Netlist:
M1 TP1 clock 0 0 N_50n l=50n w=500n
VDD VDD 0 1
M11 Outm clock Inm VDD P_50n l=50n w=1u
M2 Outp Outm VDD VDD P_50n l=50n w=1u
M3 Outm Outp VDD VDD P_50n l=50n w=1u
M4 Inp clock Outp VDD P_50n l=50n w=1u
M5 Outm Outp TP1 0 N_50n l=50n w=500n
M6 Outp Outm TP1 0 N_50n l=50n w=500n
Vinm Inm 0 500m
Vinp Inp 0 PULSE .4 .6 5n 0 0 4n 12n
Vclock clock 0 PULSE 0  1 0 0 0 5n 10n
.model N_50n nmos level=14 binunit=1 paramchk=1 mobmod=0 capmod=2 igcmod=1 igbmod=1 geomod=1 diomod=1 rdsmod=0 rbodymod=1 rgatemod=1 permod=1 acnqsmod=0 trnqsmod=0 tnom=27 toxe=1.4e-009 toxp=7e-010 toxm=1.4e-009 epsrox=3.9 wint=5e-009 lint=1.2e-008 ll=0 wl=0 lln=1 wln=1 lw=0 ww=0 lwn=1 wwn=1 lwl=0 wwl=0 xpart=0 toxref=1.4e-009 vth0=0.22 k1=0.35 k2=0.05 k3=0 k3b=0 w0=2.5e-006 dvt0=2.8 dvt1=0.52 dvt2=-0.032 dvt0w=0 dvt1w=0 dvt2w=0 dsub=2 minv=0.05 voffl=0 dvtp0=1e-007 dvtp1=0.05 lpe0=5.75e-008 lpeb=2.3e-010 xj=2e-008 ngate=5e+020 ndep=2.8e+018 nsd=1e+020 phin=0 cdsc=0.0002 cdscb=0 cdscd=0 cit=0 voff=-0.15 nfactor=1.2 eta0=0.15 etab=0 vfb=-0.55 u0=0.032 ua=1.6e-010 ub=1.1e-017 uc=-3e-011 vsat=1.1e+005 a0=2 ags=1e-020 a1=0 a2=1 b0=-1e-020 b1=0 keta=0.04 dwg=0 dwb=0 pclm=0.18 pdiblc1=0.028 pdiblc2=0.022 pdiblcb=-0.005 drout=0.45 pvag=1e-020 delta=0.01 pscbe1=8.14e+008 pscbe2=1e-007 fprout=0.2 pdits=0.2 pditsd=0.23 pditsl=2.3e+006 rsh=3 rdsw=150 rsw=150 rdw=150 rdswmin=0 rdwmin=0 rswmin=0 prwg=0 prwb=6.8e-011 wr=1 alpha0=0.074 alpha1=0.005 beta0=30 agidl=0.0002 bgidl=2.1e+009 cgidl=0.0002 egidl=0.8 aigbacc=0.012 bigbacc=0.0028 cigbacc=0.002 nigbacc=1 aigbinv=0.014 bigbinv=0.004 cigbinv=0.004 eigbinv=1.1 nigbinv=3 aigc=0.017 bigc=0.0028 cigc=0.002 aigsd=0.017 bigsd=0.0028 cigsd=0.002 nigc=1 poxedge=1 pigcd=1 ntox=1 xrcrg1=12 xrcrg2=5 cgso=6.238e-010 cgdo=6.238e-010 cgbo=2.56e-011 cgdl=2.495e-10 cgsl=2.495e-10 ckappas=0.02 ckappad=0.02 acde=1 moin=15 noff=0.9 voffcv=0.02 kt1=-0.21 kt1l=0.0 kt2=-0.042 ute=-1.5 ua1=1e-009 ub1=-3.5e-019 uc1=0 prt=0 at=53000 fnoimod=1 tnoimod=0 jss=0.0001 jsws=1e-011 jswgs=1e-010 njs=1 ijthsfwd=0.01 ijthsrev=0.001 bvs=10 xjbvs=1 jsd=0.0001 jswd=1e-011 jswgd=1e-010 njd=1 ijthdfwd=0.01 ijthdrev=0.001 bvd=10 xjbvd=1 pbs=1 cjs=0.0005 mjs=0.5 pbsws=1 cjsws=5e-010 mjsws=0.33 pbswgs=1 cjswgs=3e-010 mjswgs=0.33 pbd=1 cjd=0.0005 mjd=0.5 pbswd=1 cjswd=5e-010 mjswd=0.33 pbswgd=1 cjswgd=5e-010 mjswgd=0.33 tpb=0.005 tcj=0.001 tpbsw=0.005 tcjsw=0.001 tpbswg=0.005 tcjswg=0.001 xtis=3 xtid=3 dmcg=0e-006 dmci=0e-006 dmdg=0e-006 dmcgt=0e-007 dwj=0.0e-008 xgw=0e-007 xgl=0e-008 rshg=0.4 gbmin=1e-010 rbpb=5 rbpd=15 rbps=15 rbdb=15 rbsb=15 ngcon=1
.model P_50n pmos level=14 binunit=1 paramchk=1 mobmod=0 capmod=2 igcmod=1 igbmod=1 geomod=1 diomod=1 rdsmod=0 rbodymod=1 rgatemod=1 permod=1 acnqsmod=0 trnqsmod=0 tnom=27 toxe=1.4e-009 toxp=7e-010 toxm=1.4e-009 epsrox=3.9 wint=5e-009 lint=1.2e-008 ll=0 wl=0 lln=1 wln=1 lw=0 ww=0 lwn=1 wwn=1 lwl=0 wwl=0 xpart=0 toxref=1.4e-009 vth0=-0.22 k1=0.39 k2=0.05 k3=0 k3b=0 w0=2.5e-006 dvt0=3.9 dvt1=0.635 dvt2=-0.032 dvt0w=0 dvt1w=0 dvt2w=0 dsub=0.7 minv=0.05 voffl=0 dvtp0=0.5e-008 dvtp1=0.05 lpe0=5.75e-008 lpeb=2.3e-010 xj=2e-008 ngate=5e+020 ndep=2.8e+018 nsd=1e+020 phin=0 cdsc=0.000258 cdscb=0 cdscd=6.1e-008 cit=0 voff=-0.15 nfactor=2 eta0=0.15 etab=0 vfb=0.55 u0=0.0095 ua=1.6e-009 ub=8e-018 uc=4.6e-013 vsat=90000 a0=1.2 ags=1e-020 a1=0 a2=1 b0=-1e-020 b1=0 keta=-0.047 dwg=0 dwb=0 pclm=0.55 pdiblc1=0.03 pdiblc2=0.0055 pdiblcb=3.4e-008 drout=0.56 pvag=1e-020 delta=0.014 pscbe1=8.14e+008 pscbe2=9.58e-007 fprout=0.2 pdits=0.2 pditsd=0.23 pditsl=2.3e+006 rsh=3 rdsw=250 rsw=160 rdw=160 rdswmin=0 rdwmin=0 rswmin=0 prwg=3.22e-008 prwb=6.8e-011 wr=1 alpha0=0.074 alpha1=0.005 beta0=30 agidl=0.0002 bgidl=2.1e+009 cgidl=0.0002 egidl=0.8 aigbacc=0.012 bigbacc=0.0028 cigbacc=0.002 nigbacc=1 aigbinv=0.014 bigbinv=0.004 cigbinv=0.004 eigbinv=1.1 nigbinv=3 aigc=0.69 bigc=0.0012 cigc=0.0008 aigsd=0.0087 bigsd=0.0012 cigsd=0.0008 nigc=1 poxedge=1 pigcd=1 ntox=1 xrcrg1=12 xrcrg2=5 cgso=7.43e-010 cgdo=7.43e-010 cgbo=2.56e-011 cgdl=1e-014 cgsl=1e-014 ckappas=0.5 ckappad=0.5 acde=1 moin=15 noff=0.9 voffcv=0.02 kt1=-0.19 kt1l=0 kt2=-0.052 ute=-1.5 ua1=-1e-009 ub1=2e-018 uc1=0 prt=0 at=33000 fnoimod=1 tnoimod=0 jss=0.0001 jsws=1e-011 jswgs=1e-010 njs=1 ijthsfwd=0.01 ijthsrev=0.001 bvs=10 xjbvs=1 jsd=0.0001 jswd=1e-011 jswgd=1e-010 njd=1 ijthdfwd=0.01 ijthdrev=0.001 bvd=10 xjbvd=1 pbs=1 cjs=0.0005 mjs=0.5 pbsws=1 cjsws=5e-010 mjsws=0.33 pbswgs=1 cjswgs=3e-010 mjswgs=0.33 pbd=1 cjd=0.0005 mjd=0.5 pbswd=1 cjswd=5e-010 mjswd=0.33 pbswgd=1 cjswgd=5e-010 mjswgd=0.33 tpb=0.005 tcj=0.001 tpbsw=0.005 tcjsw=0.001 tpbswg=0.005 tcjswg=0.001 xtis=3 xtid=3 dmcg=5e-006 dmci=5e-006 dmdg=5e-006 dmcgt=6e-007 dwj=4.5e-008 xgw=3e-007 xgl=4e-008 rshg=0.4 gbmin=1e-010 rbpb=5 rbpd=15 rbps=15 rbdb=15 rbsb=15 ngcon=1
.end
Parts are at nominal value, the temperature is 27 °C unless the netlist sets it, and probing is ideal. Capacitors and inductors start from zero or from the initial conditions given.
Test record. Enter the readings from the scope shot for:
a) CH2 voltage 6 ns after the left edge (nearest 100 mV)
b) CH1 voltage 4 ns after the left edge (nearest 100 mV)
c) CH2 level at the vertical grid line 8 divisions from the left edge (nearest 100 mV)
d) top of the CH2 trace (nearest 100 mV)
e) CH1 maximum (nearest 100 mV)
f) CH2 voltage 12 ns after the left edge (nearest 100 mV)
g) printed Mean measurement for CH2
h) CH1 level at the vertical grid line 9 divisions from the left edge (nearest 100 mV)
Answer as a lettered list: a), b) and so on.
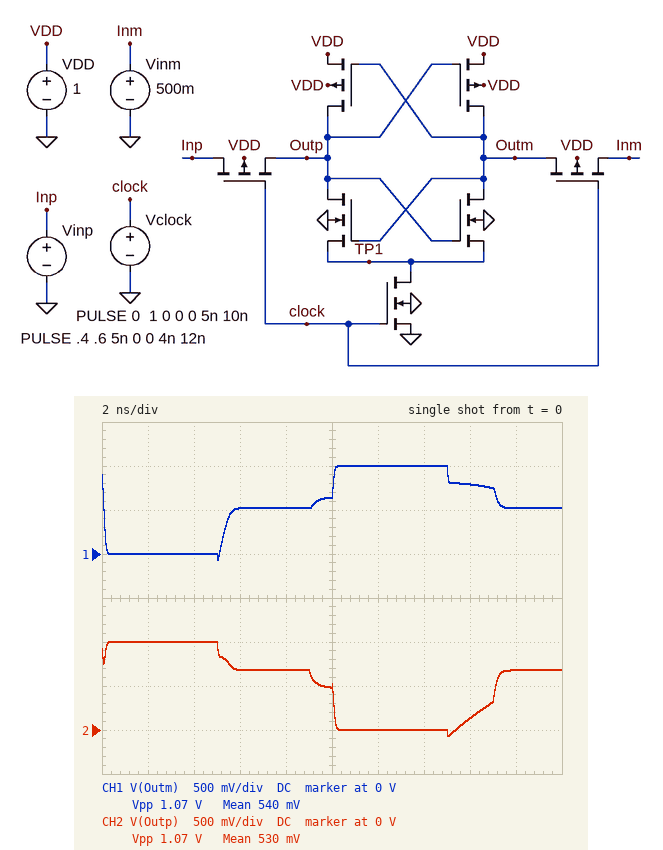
a) 700 mV
b) 0 V
c) 100 mV
d) 1.0 V
e) 1.0 V
f) 0 V
g) 530 mV
h) 500 mV
